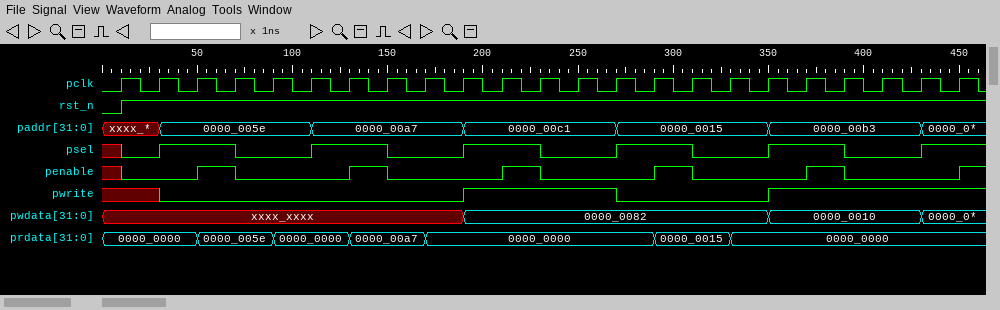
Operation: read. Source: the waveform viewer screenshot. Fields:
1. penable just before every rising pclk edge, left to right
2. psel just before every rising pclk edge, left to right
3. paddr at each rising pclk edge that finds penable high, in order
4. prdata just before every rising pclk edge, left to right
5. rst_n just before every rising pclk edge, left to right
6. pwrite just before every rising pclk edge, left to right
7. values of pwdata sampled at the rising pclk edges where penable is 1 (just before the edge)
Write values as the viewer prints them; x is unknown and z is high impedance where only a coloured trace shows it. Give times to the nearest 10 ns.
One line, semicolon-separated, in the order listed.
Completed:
x 0 0 1 0 0 0 1 0 0 0 1 0 0 0 1 0 0 0 1 0 0 0; x 0 1 1 0 0 1 1 0 0 1 1 0 0 1 1 0 0 1 1 0 0 1; 0000_005e, 0000_00a7, 0000_00c1, 0000_0015, 0000_00b3; 0000_0000, 0000_0000, 0000_0000, 0000_005e, 0000_005e, 0000_0000, 0000_0000, 0000_00a7, 0000_00a7, 0000_0000, 0000_0000, 0000_0000, 0000_0000, 0000_0000, 0000_0000, 0000_0015, 0000_0015, 0000_0000, 0000_0000, 0000_0000, 0000_0000, 0000_0000, 0000_0000; 0 1 1 1 1 1 1 1 1 1 1 1 1 1 1 1 1 1 1 1 1 1 1; x x 0 0 0 0 0 0 0 0 1 1 1 1 0 0 0 0 1 1 1 1 1; xxxx_xxxx, xxxx_xxxx, 0000_0082, 0000_0082, 0000_0010
